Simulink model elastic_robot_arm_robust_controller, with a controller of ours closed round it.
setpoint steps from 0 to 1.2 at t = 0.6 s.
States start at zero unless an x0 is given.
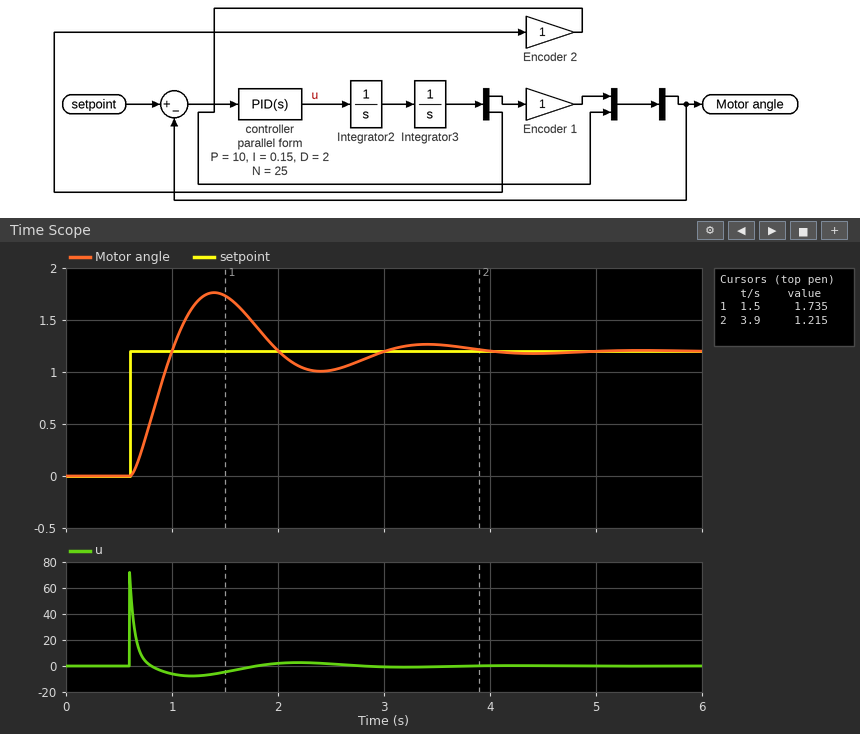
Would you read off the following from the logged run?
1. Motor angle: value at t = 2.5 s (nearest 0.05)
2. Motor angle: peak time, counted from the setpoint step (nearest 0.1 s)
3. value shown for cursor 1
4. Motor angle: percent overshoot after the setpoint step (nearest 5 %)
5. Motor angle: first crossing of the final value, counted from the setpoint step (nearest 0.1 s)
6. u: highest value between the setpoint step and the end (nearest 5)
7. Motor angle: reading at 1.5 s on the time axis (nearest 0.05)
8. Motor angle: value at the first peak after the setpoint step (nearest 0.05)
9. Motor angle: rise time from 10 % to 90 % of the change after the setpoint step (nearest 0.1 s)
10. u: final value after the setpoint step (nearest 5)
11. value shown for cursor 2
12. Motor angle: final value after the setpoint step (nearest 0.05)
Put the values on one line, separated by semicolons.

1.00; 0.8 s; 1.735; 45 %; 0.4 s; 70; 1.75; 1.75; 0.3 s; 0; 1.215; 1.20
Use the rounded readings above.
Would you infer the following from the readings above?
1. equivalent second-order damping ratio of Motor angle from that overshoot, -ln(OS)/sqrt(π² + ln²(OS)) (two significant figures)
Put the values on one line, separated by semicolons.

0.25
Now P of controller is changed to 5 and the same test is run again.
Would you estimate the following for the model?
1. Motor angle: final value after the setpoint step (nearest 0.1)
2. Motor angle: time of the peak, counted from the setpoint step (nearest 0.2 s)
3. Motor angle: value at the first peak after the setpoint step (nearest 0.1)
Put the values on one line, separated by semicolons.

1.2; 1.0 s; 1.6
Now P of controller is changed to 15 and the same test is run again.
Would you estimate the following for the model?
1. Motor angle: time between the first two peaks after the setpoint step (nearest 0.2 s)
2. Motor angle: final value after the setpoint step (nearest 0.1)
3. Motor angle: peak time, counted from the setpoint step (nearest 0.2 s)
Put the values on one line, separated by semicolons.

1.6 s; 1.2; 0.6 s
